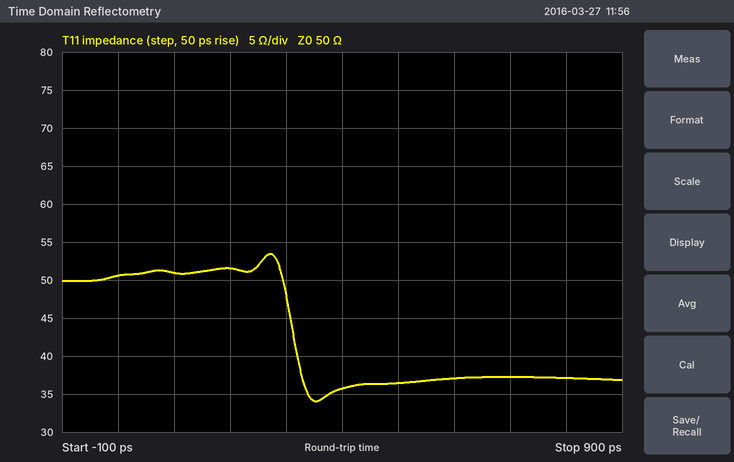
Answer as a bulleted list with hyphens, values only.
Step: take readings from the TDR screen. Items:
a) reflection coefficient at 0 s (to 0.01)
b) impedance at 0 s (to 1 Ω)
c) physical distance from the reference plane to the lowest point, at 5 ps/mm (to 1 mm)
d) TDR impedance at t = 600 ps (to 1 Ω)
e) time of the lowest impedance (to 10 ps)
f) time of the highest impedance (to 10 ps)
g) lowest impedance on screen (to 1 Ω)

- +0.01
- 51 Ω
- 35 mm
- 37 Ω
- 350 ps
- 270 ps
- 34 Ω
